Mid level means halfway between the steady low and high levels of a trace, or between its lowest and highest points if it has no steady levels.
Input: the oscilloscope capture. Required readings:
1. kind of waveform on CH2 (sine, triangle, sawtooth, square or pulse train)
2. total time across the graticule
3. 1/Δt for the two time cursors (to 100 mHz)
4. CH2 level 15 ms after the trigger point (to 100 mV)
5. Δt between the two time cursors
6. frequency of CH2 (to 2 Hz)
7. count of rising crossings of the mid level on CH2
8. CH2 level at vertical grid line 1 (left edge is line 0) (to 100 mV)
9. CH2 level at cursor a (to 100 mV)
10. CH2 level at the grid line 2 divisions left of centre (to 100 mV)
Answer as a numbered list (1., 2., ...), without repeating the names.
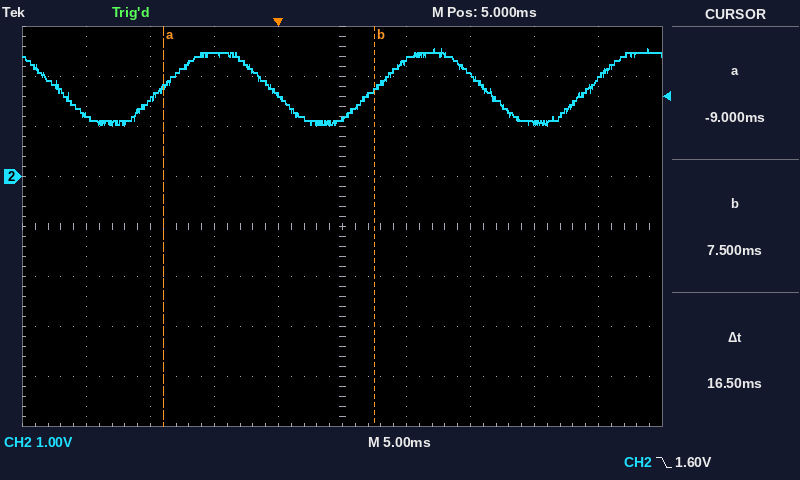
1. sine
2. 50 ms
3. 60.6 Hz
4. 2.0 V
5. 16.5 ms
6. 60 Hz
7. 3
8. 1.2 V
9. 1.8 V
10. 2.5 V
